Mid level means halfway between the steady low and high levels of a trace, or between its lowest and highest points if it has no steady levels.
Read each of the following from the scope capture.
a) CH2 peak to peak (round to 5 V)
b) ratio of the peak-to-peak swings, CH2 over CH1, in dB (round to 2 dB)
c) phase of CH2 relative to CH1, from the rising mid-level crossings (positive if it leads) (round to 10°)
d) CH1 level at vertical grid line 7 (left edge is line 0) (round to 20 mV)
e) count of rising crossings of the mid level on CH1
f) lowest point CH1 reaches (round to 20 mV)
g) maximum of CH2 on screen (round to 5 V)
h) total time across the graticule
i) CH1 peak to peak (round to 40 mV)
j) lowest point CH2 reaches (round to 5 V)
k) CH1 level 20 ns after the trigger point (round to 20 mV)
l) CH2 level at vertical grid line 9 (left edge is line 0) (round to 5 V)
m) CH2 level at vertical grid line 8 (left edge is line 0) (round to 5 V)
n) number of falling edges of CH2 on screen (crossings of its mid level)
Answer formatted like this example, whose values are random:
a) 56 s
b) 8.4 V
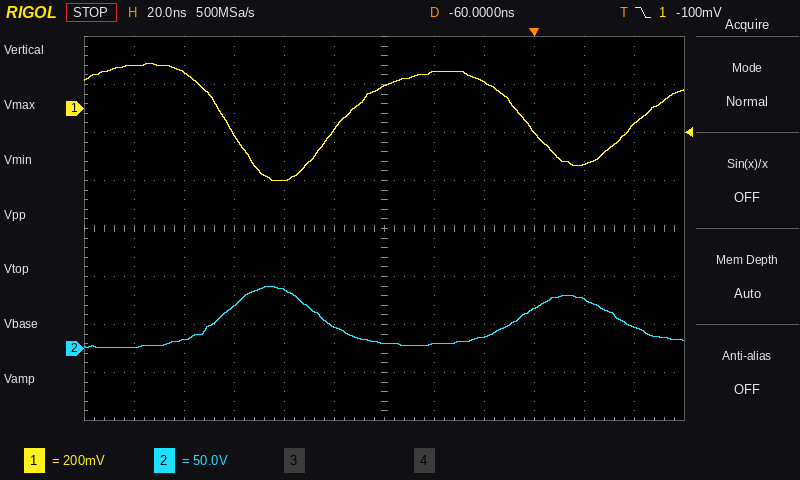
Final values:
a) 65 V
b) 42 dB
c) +140°
d) 160 mV
e) 2
f) -300 mV
g) 65 V
h) 240 ns
i) 480 mV
j) 0 V
k) -240 mV
l) 40 V
m) 10 V
n) 2
